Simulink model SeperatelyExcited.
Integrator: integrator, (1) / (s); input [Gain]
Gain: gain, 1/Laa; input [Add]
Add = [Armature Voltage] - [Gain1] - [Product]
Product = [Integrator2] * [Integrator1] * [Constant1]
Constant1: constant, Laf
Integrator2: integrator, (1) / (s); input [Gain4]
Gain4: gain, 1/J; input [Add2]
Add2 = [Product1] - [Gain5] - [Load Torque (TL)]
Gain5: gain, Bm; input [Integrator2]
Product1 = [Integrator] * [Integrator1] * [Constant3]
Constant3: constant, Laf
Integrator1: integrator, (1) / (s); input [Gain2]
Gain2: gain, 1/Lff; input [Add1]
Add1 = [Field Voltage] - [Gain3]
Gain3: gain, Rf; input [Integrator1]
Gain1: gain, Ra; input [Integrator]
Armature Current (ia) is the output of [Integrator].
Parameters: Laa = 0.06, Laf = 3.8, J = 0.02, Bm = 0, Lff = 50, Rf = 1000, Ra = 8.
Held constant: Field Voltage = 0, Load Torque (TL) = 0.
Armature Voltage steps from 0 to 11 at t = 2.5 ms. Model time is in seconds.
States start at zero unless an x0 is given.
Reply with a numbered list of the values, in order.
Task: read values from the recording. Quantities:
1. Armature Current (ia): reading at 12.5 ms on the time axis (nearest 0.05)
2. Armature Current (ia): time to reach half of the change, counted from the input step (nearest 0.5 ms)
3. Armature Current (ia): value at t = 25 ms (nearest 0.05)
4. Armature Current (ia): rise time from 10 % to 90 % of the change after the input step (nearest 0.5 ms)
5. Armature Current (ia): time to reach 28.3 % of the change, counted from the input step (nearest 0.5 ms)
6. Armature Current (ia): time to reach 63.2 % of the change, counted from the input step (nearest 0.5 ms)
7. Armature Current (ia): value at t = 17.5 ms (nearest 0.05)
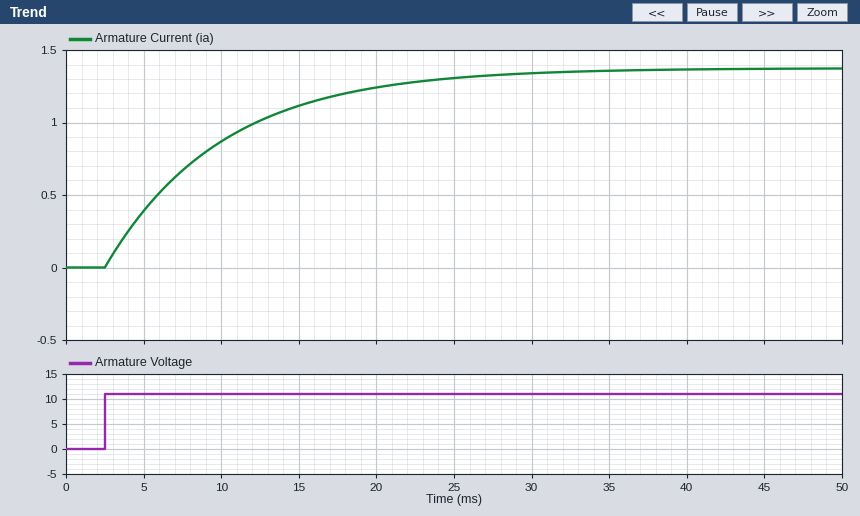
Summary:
1. 1.00
2. 5.0 ms
3. 1.30
4. 16.5 ms
5. 2.5 ms
6. 7.5 ms
7. 1.20
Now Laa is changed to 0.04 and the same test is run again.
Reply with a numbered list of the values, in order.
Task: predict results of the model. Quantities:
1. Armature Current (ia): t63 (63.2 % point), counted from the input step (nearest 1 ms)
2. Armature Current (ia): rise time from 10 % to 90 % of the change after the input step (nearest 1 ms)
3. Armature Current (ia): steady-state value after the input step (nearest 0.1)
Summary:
1. 5 ms
2. 11 ms
3. 1.4
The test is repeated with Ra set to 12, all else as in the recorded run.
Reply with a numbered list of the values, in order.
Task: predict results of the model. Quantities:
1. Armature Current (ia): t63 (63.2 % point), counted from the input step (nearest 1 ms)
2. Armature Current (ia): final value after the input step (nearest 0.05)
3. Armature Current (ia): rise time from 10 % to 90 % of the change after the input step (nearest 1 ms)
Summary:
1. 5 ms
2. 0.90
3. 11 ms
